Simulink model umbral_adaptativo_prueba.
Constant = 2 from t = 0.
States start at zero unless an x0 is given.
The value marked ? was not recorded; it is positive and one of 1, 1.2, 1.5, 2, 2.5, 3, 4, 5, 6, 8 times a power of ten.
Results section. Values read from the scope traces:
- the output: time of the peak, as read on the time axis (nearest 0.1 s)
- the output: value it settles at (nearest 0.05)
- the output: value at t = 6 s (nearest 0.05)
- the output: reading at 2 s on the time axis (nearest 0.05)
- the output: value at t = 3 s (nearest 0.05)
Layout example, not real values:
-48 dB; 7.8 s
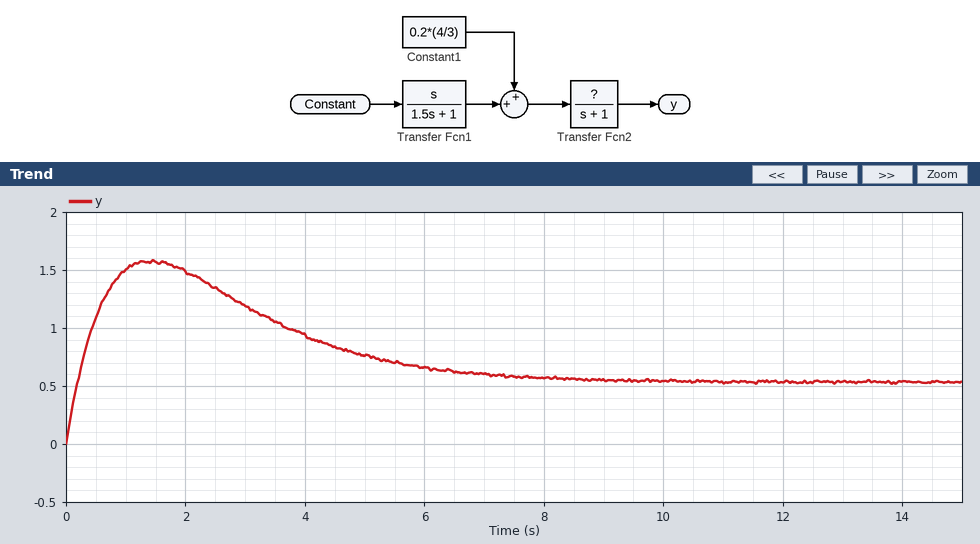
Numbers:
1.4 s; 0.55; 0.65; 1.50; 1.20
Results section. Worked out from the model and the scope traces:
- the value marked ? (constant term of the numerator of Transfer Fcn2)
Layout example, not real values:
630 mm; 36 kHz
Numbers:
2
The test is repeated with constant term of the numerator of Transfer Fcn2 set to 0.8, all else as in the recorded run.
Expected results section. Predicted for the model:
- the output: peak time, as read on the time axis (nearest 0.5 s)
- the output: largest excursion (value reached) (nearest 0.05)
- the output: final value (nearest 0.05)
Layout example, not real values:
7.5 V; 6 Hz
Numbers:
1.5 s; 0.65; 0.20
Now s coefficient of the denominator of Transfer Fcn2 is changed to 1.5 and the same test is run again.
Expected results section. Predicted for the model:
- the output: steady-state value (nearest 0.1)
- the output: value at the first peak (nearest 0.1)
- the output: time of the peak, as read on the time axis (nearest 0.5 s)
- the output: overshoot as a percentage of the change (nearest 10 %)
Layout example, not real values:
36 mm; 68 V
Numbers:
0.5; 1.3; 2.0 s; 150 %
